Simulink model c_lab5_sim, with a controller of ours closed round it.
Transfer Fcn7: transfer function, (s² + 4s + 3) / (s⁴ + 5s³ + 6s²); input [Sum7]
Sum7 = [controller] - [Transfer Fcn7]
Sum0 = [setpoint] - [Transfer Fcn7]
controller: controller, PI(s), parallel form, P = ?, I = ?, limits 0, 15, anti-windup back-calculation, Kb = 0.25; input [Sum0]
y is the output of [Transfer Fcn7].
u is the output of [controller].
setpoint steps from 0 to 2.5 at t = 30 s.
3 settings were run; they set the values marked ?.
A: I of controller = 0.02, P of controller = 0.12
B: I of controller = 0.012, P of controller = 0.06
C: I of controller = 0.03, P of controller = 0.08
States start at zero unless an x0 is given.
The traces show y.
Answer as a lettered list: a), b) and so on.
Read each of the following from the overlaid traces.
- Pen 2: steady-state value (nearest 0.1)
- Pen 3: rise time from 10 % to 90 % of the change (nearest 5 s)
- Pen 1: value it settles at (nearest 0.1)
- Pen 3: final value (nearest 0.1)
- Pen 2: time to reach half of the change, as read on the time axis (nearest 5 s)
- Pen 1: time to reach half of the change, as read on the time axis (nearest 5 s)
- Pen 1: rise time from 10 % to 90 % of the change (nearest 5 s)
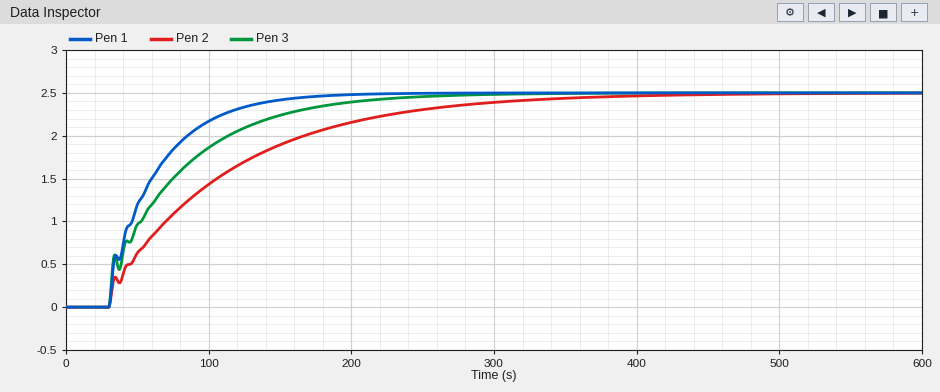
a) 2.5
b) 120 s
c) 2.5
d) 2.5
e) 85 s
f) 50 s
g) 80 s
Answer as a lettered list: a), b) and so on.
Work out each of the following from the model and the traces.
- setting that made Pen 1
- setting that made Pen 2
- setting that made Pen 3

a) C
b) B
c) A
